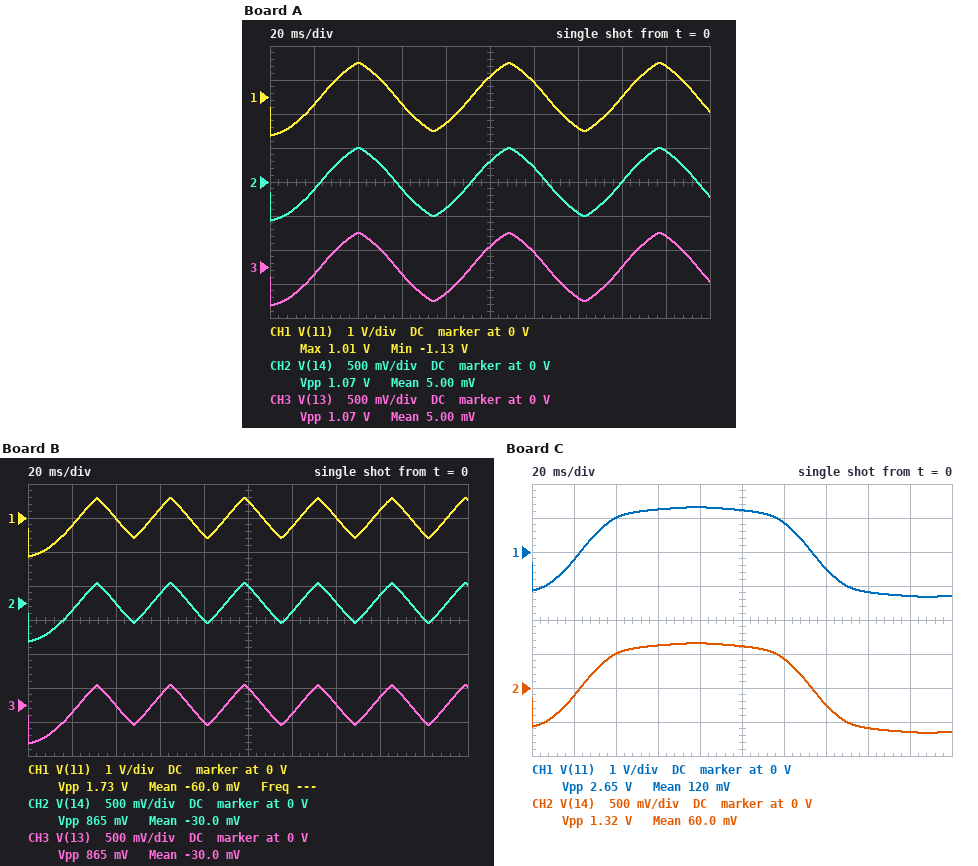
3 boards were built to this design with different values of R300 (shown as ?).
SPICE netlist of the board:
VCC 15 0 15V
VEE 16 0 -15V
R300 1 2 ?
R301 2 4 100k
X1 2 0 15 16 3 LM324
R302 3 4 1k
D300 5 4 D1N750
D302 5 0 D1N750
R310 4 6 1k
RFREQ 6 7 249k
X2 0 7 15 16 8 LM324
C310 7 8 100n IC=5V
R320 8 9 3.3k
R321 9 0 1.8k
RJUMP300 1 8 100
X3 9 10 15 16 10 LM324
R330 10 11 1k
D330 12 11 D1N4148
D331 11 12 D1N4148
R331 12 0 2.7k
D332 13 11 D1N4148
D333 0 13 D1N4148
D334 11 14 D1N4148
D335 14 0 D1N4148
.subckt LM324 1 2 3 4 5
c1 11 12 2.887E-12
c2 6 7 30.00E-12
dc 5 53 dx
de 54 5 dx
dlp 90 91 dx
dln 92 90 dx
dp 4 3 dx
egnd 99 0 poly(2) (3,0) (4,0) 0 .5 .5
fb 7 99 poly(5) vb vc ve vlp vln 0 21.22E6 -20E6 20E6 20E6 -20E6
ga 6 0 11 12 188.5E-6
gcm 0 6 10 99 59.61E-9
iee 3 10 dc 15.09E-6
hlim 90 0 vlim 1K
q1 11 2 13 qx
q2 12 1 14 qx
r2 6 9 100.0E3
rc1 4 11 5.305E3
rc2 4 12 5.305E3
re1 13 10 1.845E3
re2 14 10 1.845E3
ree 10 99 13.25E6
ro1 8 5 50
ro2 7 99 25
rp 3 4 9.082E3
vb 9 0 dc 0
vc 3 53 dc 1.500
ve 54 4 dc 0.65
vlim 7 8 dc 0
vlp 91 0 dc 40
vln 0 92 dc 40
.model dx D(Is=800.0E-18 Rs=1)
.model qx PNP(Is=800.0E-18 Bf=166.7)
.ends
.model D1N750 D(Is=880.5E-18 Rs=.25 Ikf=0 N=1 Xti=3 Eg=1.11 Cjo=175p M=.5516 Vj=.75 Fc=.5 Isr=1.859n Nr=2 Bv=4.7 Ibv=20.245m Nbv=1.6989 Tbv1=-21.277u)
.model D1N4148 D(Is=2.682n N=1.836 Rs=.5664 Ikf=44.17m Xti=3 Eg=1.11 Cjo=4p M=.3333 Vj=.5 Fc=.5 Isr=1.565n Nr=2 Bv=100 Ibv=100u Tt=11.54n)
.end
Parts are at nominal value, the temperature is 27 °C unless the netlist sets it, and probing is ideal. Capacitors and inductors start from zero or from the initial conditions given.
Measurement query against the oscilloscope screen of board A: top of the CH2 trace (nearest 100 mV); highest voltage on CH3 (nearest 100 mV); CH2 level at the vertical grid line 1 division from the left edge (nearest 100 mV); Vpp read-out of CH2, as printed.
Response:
500 mV
500 mV
-100 mV
1.07 V
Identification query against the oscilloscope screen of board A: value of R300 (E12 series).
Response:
68 kΩ
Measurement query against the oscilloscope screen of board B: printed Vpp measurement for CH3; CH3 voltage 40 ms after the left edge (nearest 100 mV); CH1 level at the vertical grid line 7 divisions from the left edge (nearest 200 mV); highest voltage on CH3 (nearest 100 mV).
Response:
865 mV
0 V
0 V
300 mV
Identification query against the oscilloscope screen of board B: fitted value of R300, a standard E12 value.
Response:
33 kΩ
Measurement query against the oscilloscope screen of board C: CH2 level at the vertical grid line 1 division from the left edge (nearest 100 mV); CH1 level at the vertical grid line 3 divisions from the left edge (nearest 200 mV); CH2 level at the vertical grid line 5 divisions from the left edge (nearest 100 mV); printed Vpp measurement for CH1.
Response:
-100 mV
1.2 V
600 mV
2.65 V
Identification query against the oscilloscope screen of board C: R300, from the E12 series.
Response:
220 kΩ
